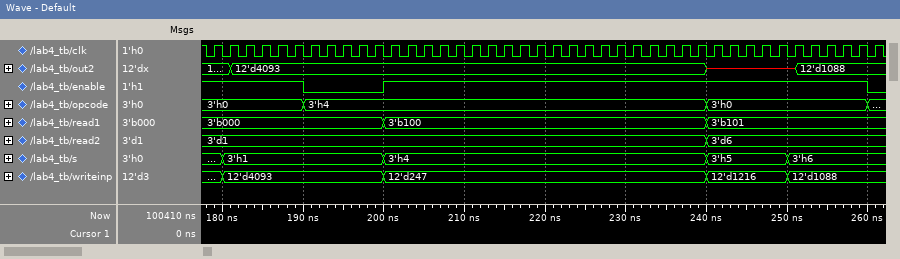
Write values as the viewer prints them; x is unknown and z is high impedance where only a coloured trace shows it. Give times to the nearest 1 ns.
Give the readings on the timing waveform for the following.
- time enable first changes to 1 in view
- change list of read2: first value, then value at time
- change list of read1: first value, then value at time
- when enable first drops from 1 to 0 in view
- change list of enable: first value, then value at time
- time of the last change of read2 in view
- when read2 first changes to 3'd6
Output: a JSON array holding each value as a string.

["200 ns", "3'd1, 3'd6 at 240 ns", "3'b000, 3'b100 at 200 ns, 3'b101 at 240 ns", "190 ns", "1, 0 at 190 ns, 1 at 200 ns, 0 at 260 ns", "240 ns", "240 ns"]
